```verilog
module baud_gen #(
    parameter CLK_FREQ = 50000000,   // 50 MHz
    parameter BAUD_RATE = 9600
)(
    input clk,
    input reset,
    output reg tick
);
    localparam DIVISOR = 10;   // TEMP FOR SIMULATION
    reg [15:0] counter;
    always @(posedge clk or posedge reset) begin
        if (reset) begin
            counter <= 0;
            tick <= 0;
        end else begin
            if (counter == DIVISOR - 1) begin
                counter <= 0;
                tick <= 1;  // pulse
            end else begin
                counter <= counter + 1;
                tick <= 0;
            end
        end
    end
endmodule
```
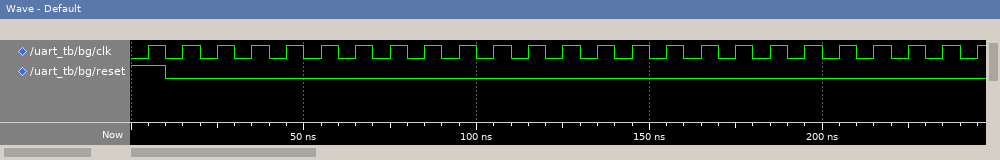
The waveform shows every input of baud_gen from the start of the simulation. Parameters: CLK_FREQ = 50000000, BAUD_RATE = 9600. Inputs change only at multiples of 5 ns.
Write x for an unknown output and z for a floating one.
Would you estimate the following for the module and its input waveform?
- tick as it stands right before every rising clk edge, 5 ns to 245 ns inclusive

0 0 0 0 0 0 0 0 0 0 0 1 0 0 0 0 0 0 0 0 0 1 0 0 0
